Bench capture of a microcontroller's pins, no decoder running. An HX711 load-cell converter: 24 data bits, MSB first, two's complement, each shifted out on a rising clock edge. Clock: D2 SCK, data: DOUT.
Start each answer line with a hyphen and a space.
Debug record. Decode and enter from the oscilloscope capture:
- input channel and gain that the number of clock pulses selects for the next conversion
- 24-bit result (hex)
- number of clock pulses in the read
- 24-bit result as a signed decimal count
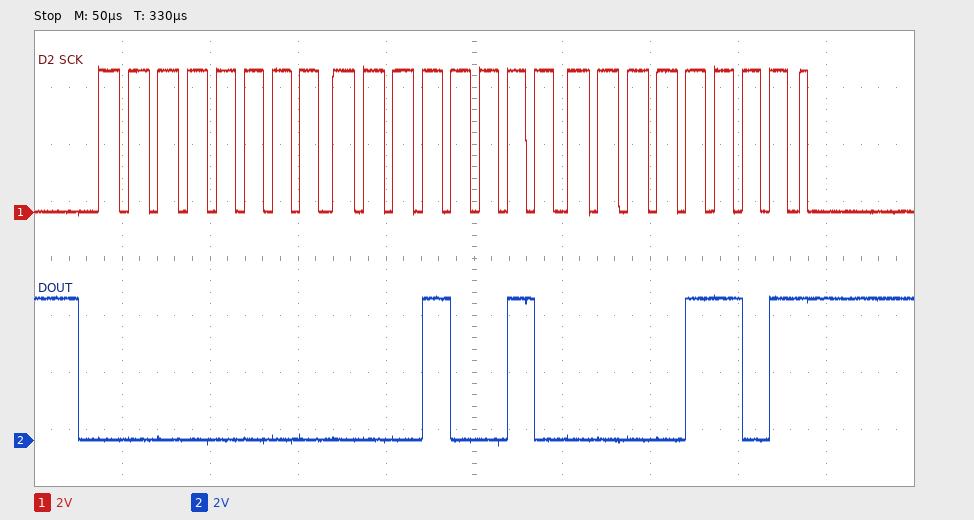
- channel A, gain 128
- 0x00120D
- 25
- 4621
